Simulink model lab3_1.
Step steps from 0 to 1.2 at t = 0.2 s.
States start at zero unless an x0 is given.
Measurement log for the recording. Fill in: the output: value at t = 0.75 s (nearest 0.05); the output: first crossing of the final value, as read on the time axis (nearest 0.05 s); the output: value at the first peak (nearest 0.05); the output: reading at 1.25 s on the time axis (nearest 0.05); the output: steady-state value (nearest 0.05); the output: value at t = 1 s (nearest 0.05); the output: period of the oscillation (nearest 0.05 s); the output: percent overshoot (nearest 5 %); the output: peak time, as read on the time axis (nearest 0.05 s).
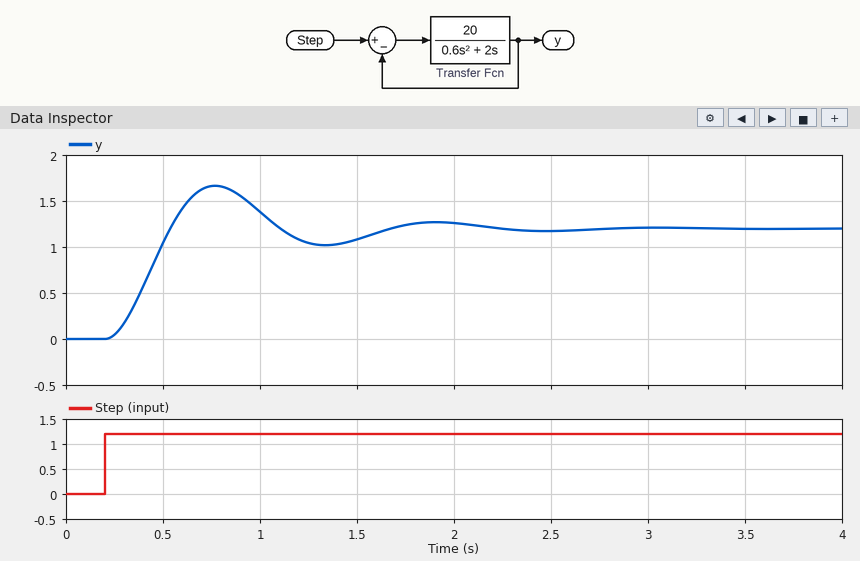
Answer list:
1.65
0.55 s
1.65
1.05
1.20
1.40
1.15 s
40 %
0.75 s
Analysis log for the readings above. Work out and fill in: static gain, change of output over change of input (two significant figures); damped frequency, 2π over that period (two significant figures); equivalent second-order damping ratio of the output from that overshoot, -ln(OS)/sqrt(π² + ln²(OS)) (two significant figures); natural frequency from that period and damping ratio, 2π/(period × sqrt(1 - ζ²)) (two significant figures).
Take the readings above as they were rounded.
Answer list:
1.0
5.5 rad/s
0.28
5.7 rad/s
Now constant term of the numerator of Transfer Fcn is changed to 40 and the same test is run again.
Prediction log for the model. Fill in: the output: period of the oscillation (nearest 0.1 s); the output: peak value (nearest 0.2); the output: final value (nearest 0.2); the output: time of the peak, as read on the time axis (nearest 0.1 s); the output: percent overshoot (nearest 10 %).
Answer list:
0.8 s
1.8
1.2
0.6 s
50 %
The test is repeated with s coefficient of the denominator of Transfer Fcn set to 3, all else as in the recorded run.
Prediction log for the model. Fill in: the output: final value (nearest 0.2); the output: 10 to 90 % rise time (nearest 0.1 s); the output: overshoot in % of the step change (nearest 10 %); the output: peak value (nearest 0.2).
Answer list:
1.2
0.3 s
20 %
1.4
